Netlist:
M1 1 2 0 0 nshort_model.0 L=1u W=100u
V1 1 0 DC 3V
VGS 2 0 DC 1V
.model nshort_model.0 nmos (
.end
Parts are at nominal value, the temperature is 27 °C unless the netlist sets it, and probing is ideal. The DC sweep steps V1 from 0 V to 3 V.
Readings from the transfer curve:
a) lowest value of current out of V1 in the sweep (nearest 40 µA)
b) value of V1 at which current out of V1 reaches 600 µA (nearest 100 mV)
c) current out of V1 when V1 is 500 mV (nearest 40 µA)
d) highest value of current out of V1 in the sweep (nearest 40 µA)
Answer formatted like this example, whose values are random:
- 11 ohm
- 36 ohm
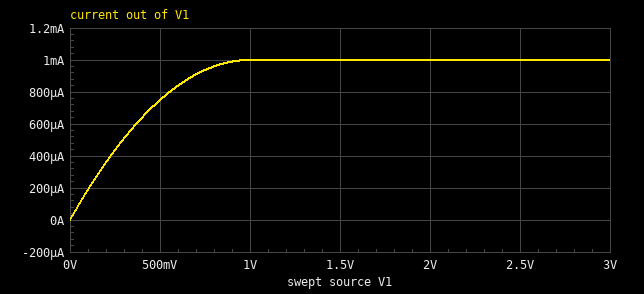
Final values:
- 0 A
- 400 mV
- 760 µA
- 1.00 mA
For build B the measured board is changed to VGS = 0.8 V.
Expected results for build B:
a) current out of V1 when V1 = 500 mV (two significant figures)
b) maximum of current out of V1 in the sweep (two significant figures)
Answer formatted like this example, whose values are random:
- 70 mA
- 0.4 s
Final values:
- 550 µA
- 640 µA
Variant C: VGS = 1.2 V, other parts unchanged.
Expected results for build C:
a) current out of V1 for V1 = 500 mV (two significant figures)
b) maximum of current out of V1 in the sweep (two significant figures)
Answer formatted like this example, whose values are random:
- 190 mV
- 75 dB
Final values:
- 950 µA
- 1.4 mA
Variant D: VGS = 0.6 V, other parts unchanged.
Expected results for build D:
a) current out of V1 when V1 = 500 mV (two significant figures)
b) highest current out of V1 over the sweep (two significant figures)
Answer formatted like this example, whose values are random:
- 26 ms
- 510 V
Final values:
- 350 µA
- 360 µA
